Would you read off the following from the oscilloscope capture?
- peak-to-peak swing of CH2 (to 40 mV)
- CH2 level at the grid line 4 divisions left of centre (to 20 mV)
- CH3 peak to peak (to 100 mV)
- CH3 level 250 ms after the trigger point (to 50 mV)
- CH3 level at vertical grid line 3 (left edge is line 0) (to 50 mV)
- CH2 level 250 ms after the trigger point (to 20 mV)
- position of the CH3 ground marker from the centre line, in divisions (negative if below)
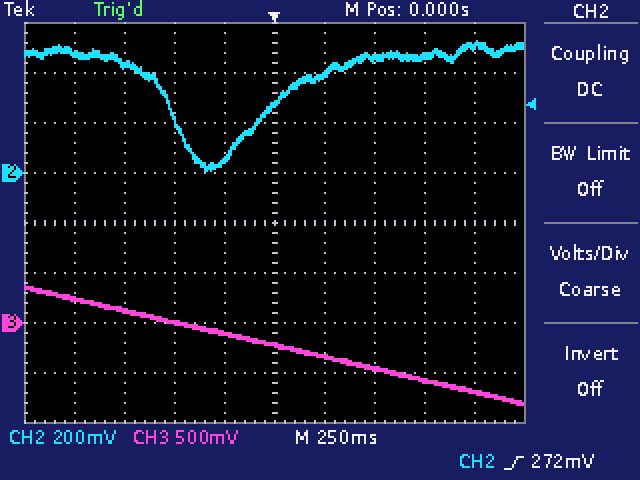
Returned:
520 mV
480 mV
1.20 V
-350 mV
0 mV
400 mV
-2.0 div
